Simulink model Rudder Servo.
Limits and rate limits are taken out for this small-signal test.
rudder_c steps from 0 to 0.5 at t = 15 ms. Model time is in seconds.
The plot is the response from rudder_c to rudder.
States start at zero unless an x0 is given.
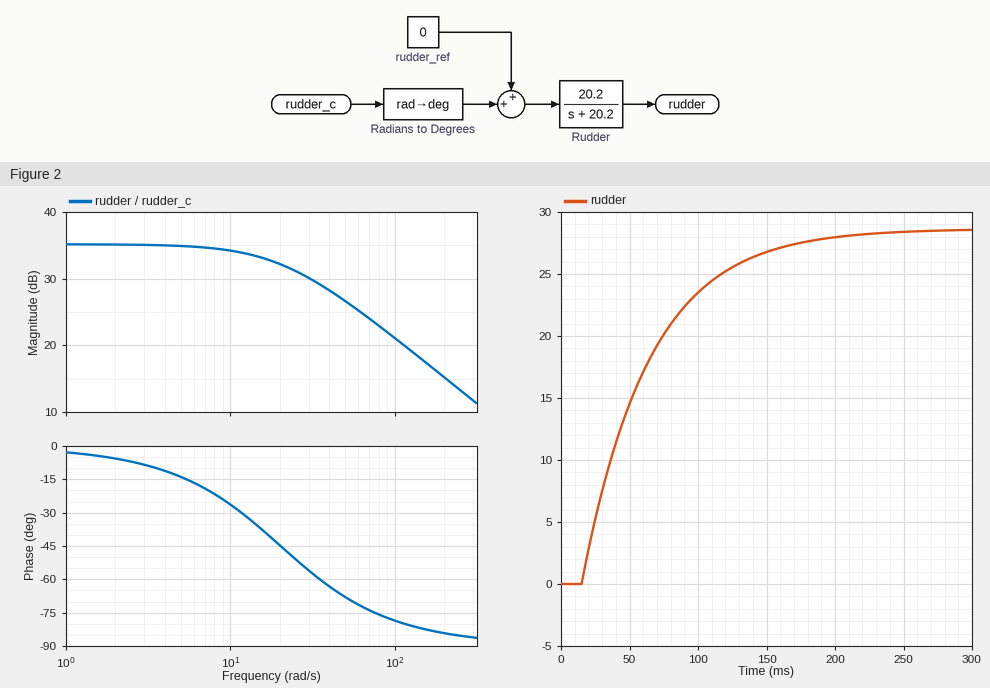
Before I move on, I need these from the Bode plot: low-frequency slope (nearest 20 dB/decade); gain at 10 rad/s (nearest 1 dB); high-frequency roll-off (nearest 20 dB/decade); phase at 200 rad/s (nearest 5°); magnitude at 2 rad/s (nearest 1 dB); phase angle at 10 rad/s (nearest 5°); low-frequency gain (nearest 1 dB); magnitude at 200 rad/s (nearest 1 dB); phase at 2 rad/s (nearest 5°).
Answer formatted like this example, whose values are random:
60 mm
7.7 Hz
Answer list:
0 dB/decade
34 dB
-20 dB/decade
-85°
35 dB
-25°
35 dB
15 dB
-5°
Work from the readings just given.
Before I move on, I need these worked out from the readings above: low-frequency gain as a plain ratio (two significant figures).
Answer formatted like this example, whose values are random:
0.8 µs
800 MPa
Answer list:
56
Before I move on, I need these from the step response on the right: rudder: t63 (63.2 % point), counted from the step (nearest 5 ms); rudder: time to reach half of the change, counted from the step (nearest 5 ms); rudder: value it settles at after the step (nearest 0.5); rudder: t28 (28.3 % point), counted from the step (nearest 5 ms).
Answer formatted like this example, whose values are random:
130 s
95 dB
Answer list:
50 ms
35 ms
28.5
15 ms
